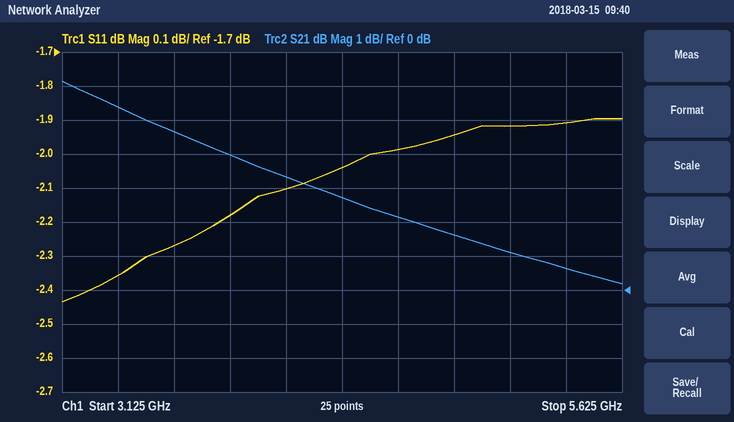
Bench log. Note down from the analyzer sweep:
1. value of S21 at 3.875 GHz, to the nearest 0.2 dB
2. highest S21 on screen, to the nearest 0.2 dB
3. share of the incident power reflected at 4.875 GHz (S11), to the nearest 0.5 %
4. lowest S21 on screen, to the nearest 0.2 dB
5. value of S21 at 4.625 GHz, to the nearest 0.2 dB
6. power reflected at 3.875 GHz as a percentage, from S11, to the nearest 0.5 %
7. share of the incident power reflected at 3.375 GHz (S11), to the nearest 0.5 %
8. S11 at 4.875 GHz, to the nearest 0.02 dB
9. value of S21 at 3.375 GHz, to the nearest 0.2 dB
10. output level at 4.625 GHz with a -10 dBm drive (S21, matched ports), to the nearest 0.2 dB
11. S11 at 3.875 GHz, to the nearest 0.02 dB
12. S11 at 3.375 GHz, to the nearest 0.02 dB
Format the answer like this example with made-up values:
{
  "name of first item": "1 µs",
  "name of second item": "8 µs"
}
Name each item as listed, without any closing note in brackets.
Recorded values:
{
  "value of S21 at 3.875 GHz, to the nearest 0.2 dB": "4.0 dB",
  "highest S21 on screen, to the nearest 0.2 dB": "6.2 dB",
  "share of the incident power reflected at 4.875 GHz (S11), to the nearest 0.5 %": "64.0 %",
  "lowest S21 on screen, to the nearest 0.2 dB": "0.2 dB",
  "value of S21 at 4.625 GHz, to the nearest 0.2 dB": "2.2 dB",
  "power reflected at 3.875 GHz as a percentage, from S11, to the nearest 0.5 %": "60.5 %",
  "share of the incident power reflected at 3.375 GHz (S11), to the nearest 0.5 %": "58.0 %",
  "S11 at 4.875 GHz, to the nearest 0.02 dB": "-1.94 dB",
  "value of S21 at 3.375 GHz, to the nearest 0.2 dB": "5.4 dB",
  "output level at 4.625 GHz with a -10 dBm drive (S21, matched ports), to the nearest 0.2 dB": "-7.8 dBm",
  "S11 at 3.875 GHz, to the nearest 0.02 dB": "-2.18 dB",
  "S11 at 3.375 GHz, to the nearest 0.02 dB": "-2.36 dB"
}
